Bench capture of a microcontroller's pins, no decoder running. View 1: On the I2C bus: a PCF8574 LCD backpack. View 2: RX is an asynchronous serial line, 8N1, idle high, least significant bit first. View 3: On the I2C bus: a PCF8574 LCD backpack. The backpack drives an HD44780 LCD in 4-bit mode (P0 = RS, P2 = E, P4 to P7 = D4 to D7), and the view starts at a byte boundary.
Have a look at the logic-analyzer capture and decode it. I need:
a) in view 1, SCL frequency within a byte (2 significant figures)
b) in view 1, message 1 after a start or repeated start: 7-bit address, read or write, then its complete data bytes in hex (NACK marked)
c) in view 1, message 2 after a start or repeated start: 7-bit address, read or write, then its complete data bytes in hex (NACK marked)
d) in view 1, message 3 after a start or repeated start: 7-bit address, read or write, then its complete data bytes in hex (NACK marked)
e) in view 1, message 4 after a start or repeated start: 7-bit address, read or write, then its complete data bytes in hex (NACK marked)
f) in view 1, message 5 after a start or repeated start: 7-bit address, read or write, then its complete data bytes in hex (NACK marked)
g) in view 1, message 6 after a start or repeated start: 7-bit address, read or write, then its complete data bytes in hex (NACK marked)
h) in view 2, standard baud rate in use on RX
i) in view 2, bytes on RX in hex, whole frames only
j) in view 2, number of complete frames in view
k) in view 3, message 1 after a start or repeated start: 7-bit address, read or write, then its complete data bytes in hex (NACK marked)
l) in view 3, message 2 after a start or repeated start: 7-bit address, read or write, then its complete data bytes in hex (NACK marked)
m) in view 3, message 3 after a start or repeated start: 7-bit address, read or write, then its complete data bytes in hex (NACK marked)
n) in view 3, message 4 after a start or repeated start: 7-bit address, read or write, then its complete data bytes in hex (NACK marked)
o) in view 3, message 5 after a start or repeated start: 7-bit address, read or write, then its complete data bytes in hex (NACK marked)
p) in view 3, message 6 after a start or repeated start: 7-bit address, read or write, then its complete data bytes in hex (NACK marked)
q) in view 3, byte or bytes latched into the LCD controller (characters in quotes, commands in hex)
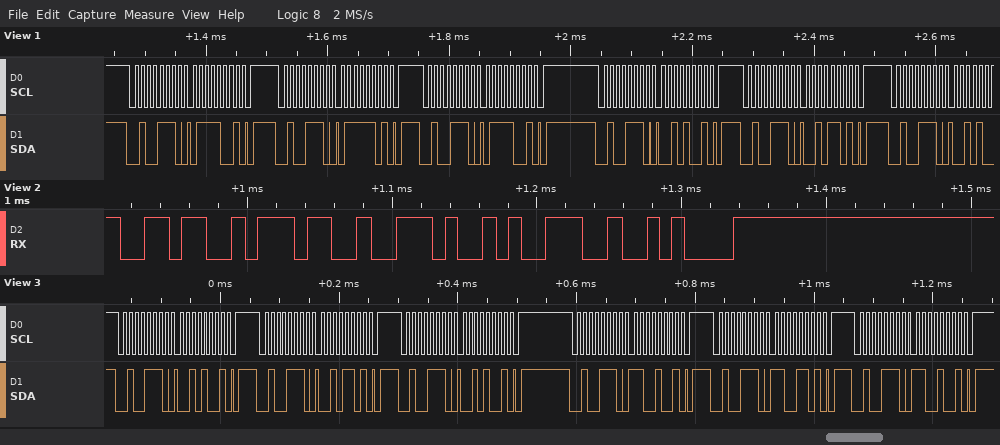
100 kHz
0x27 write: 79
0x27 write: 7D
0x27 write: 79
0x27 write: 29
0x27 write: 2D
0x27 write
115200 baud
0x36 0x37 0x2E 0x39 0x0A
5
0x27 write: 29
0x27 write: 2D
0x27 write: 29
0x27 write: C9
0x27 write: CD
0x27 write: C9
','
